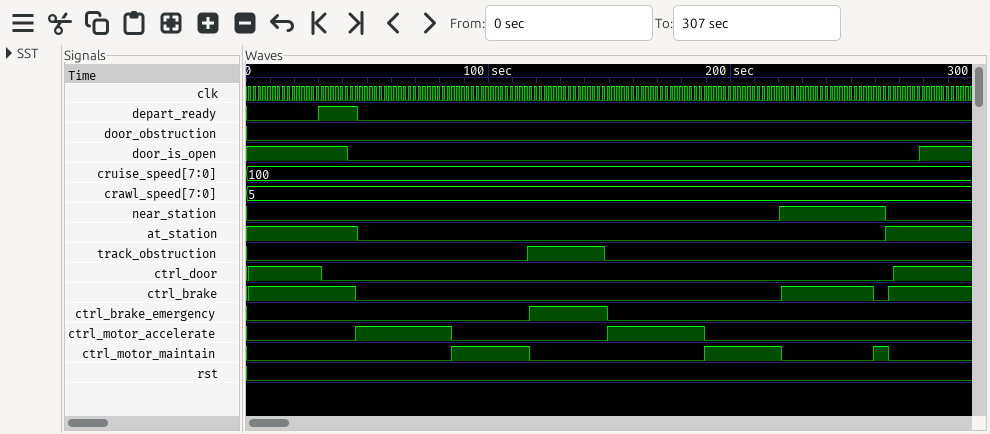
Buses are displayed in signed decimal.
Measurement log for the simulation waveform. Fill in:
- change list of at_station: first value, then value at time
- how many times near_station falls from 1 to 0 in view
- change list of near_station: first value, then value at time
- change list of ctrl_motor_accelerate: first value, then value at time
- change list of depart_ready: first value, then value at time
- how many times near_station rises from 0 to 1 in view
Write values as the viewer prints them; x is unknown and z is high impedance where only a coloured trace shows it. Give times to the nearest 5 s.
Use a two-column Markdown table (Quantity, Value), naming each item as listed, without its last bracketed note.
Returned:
| Quantity | Value |
|---|---|
| change list of at_station: first value, then value at time | 1, 0 at 45 s, 1 at 265 s |
| how many times near_station falls from 1 to 0 in view | 1 |
| change list of near_station: first value, then value at time | 0, 1 at 220 s, 0 at 265 s |
| change list of ctrl_motor_accelerate: first value, then value at time | 0, 1 at 45 s, 0 at 85 s, 1 at 150 s, 0 at 190 s |
| change list of depart_ready: first value, then value at time | 0, 1 at 30 s, 0 at 45 s |
| how many times near_station rises from 0 to 1 in view | 1 |
